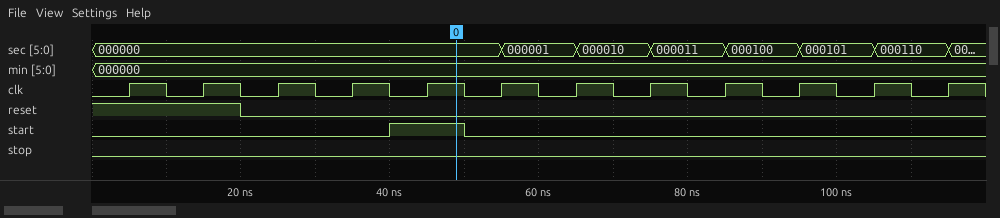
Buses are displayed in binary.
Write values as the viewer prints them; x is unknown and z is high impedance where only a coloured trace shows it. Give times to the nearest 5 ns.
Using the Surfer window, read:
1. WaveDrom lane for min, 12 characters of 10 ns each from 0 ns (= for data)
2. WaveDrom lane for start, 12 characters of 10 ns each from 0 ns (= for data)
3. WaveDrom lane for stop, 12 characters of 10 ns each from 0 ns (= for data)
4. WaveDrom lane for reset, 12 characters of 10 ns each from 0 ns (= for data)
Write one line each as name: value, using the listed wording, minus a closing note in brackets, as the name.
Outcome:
WaveDrom lane for min, 12 characters of 10 ns each from 0 ns: {name: 'min', wave: '=...........', data: '000000'}
WaveDrom lane for start, 12 characters of 10 ns each from 0 ns: {name: 'start', wave: '0...10......'}
WaveDrom lane for stop, 12 characters of 10 ns each from 0 ns: {name: 'stop', wave: '0...........'}
WaveDrom lane for reset, 12 characters of 10 ns each from 0 ns: {name: 'reset', wave: '1.0.........'}
